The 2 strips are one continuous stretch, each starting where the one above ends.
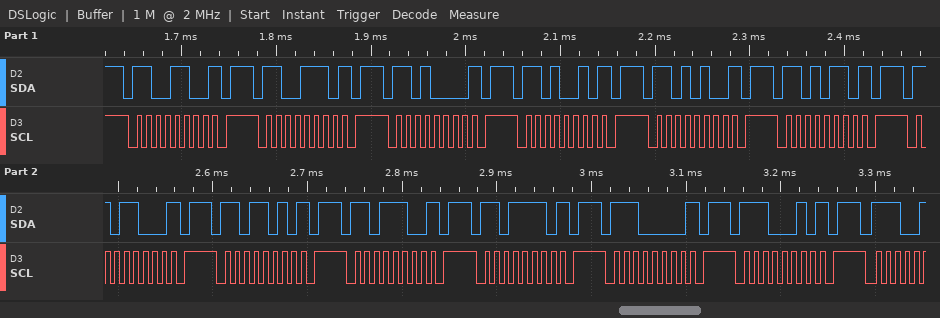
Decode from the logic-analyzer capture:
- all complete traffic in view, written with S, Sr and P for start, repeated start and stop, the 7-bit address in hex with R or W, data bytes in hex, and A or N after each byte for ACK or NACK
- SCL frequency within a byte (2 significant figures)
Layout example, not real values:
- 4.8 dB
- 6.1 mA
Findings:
- S 66W N P S 67W N P S 68W N P S 69W N P S 6AW N P S 6BW N P S 6CW N P S 6DW N P S 6EW N P S 6FW N P S 70W N P S 71W N P
- 100 kHz
